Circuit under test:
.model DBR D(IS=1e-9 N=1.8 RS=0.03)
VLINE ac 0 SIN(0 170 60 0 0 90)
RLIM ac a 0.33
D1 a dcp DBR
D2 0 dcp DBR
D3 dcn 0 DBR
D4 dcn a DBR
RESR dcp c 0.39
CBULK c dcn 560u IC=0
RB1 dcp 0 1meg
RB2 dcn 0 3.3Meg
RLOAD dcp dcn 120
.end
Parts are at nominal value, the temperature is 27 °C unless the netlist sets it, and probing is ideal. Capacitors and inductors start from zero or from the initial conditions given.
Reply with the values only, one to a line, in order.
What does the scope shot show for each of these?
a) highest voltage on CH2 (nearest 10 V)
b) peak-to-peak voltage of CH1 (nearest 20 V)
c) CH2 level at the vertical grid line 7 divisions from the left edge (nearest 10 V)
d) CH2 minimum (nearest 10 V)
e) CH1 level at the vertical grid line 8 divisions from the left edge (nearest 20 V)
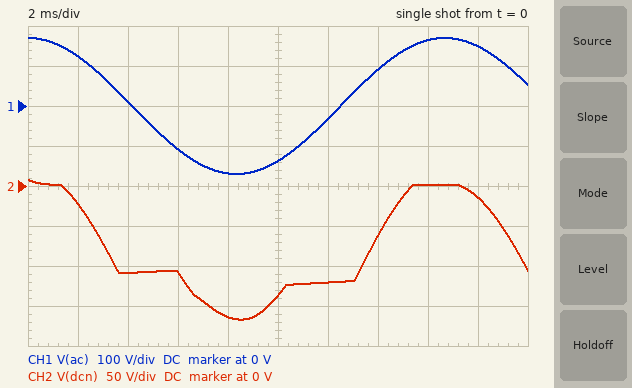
10 V
340 V
-60 V
-170 V
160 V
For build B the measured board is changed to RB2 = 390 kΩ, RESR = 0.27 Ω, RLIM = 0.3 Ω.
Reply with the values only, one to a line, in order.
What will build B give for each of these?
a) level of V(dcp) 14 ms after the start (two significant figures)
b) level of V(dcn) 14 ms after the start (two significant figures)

110 V
-43 V
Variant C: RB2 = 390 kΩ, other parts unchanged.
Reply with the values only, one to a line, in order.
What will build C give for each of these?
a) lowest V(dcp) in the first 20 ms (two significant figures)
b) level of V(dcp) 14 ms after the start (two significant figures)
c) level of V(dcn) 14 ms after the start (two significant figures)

-1.5 V
110 V
-43 V
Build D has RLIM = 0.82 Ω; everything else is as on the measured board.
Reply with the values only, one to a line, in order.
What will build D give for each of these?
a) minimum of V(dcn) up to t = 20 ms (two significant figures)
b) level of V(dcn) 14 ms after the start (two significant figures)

-160 V
-59 V
